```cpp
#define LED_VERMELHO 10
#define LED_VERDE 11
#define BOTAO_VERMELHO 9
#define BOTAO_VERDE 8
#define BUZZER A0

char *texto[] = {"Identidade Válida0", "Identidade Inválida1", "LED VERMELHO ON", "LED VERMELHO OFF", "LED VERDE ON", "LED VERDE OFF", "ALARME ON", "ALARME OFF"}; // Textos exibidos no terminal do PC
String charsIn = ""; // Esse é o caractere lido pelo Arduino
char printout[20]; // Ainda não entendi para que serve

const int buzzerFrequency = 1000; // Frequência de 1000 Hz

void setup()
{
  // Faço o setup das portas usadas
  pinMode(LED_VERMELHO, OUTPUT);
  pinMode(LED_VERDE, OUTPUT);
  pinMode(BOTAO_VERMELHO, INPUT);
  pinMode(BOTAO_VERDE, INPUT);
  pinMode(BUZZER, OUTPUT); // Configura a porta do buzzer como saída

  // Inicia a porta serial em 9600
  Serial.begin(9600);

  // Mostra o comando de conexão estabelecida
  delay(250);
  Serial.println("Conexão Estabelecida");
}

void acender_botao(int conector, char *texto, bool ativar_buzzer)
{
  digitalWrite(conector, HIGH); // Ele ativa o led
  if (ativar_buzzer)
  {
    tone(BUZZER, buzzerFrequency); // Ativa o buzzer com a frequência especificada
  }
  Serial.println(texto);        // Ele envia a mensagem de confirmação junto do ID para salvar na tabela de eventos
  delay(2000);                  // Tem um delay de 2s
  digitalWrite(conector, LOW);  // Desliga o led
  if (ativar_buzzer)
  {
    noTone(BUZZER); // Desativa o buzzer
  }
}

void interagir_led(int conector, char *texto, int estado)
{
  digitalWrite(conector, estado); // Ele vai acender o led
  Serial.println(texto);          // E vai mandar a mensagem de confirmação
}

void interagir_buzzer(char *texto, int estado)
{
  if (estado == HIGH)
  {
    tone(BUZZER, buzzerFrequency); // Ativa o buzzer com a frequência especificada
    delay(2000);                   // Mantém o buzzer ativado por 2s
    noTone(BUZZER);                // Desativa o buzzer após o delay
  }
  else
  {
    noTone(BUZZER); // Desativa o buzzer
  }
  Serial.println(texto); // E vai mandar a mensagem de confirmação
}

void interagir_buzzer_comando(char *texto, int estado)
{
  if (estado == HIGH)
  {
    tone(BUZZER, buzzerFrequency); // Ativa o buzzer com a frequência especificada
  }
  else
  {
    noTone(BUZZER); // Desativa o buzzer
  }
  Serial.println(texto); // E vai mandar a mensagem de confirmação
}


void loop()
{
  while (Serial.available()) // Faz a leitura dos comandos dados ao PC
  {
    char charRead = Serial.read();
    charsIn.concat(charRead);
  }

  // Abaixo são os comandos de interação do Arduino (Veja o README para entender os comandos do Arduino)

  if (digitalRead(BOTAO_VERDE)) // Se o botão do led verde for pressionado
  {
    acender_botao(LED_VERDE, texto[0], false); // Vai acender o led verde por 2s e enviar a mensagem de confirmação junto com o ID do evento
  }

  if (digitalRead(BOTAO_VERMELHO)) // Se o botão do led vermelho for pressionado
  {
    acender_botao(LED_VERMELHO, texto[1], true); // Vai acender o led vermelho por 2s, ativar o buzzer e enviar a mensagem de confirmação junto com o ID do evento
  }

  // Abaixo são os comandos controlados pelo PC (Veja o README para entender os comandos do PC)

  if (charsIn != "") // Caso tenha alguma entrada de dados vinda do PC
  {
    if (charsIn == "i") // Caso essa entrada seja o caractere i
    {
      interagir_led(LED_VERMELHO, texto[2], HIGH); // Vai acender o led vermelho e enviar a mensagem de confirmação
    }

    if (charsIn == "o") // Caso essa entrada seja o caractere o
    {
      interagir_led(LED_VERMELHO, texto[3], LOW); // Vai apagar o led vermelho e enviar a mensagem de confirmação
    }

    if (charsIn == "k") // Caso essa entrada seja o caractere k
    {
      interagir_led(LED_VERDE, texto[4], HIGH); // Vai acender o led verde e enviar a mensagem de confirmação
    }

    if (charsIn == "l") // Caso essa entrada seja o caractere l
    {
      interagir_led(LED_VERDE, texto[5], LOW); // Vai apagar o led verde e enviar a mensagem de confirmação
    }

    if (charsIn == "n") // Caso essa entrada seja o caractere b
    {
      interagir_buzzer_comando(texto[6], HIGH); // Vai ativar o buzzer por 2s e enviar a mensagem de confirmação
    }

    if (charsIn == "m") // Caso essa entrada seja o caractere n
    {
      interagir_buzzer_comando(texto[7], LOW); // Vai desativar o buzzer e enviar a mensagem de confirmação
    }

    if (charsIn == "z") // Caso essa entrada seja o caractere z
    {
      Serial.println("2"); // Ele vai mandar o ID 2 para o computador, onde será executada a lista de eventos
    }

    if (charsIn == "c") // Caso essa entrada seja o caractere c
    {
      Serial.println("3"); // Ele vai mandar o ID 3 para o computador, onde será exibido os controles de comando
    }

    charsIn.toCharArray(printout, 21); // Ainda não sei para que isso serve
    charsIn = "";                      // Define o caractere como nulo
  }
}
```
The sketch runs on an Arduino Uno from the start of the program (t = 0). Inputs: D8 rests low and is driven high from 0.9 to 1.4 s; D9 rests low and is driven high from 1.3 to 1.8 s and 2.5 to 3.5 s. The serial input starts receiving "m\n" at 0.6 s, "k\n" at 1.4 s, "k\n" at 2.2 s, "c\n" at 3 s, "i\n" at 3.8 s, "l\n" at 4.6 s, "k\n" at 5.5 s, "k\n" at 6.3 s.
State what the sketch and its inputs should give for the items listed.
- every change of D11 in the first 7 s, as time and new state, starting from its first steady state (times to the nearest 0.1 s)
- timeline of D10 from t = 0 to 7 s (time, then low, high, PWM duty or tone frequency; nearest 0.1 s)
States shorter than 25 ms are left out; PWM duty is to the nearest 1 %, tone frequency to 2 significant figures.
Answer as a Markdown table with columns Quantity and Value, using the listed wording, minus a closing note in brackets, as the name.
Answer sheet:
| Quantity | Value |
|---|---|
| every change of D11 in the first 7 s, as time and new state, starting from its first steady state | 0 s low; 0.9 s high; 2.9 s low; 5.5 s high |
| timeline of D10 from t = 0 to 7 s | 0 s low; 2.9 s high; 4.9 s low |
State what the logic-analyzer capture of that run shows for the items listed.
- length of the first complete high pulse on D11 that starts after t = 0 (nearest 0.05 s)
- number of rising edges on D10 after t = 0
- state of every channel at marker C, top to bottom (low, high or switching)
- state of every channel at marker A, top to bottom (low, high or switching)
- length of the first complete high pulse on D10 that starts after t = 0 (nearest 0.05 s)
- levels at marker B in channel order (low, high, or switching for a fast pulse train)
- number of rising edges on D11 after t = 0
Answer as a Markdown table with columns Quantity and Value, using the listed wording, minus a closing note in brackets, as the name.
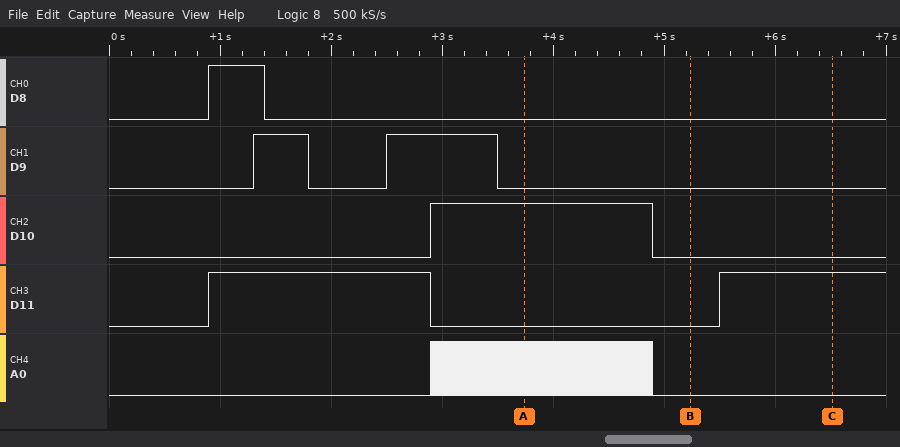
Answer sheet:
| Quantity | Value |
|---|---|
| length of the first complete high pulse on D11 that starts after t = 0 | 2.00 s |
| number of rising edges on D10 after t = 0 | 1 |
| state of every channel at marker C, top to bottom | D8 low, D9 low, D10 low, D11 high, A0 low |
| state of every channel at marker A, top to bottom | D8 low, D9 low, D10 high, D11 low, A0 switching |
| length of the first complete high pulse on D10 that starts after t = 0 | 2.00 s |
| levels at marker B in channel order | D8 low, D9 low, D10 low, D11 low, A0 low |
| number of rising edges on D11 after t = 0 | 2 |
